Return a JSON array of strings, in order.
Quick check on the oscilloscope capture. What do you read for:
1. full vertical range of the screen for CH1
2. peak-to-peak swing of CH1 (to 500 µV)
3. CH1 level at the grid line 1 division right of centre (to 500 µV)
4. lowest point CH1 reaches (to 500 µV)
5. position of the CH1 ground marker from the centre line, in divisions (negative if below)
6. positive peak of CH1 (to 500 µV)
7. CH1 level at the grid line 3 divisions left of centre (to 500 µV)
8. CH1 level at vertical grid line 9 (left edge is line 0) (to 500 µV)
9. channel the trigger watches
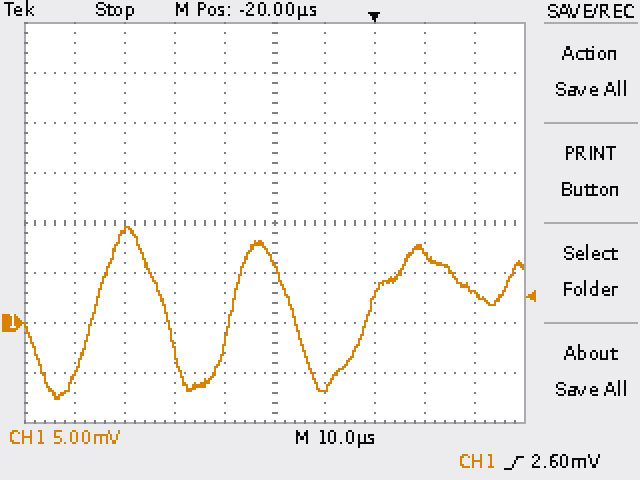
["40 mV", "17.0 mV", "-6.5 mV", "-7.5 mV", "-2.0 div", "9.5 mV", "9.0 mV", "3.0 mV", "CH1"]
